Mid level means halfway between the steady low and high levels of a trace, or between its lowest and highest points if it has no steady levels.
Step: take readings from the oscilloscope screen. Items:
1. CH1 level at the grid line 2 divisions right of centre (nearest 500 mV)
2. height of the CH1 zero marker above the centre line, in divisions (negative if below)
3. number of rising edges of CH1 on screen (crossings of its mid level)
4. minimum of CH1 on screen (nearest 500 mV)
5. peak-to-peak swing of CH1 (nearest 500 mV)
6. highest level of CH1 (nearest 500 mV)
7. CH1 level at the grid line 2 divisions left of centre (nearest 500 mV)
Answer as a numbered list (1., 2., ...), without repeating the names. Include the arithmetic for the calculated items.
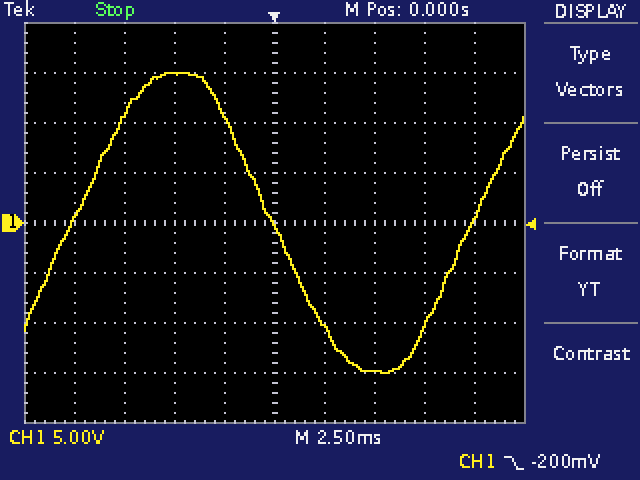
1. -15.0 V
2. 0.0 div
3. 2
4. -15.0 V
5. 15.0 V − (-15.0 V) = 30.0 V
6. 15.0 V
7. 15.0 V
